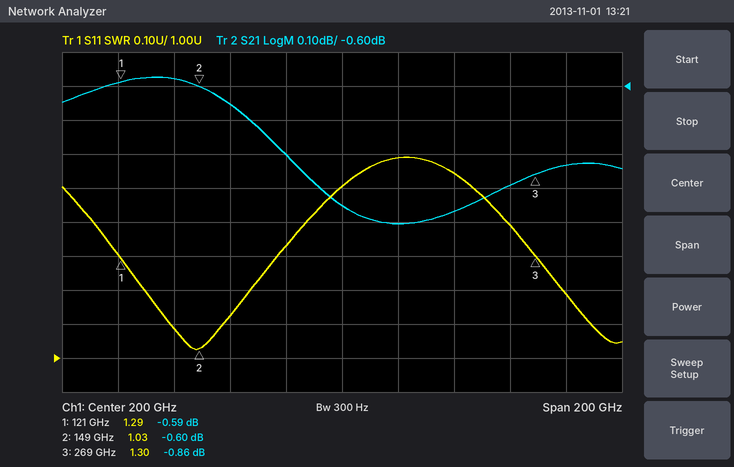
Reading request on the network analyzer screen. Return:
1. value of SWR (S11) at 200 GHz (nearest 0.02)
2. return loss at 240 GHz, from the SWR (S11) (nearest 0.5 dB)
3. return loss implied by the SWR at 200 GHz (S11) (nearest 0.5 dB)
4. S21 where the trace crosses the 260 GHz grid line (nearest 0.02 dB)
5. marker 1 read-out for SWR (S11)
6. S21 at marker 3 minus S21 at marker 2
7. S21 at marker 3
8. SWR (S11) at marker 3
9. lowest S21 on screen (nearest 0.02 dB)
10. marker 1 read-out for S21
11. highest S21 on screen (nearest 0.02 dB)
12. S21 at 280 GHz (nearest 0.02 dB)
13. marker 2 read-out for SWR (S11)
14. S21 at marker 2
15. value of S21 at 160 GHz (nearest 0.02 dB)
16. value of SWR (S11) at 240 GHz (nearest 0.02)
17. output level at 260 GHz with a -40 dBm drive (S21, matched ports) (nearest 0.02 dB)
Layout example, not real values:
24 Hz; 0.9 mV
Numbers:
1.50; 13.5 dB; 14.0 dB; -0.90 dB; 1.29; -0.26 dB; -0.86 dB; 1.30; -1.00 dB; -0.59 dB; -0.58 dB; -0.84 dB; 1.03; -0.60 dB; -0.66 dB; 1.54; -40.90 dBm
